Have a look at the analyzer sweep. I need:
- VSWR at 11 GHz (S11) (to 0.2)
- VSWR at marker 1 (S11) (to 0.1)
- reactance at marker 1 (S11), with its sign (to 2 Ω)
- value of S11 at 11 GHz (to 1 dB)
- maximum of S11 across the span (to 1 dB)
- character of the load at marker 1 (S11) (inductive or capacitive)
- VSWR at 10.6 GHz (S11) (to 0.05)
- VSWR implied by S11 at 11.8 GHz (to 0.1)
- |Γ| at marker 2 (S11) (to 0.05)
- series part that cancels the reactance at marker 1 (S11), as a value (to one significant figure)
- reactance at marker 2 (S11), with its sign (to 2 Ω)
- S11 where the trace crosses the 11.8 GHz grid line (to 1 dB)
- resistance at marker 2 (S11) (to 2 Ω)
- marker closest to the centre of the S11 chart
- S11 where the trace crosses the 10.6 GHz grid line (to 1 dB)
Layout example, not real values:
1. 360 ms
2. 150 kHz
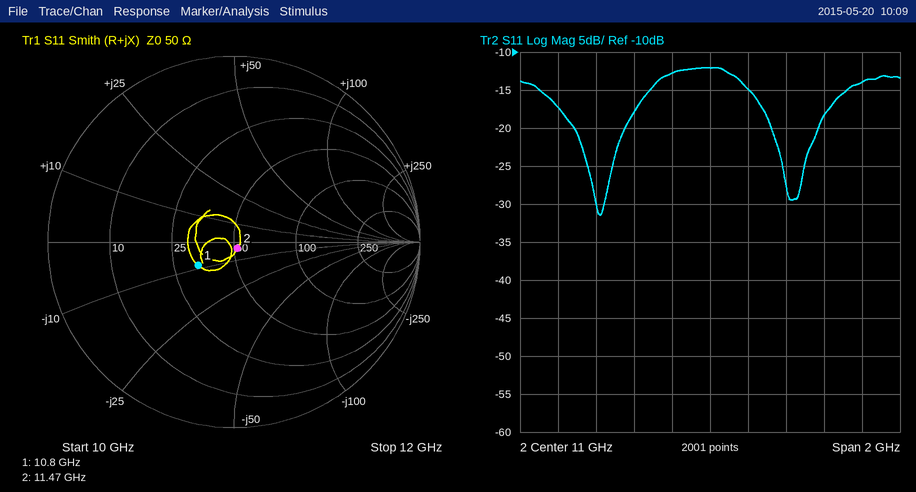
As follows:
1. 1.6
2. 1.6
3. -8 Ω
4. -12 dB
5. -12 dB
6. capacitive
7. 1.30
8. 1.5
9. 0.05
10. 100 pH
11. -4 Ω
12. -14 dB
13. 52 Ω
14. marker 2
15. -18 dB
